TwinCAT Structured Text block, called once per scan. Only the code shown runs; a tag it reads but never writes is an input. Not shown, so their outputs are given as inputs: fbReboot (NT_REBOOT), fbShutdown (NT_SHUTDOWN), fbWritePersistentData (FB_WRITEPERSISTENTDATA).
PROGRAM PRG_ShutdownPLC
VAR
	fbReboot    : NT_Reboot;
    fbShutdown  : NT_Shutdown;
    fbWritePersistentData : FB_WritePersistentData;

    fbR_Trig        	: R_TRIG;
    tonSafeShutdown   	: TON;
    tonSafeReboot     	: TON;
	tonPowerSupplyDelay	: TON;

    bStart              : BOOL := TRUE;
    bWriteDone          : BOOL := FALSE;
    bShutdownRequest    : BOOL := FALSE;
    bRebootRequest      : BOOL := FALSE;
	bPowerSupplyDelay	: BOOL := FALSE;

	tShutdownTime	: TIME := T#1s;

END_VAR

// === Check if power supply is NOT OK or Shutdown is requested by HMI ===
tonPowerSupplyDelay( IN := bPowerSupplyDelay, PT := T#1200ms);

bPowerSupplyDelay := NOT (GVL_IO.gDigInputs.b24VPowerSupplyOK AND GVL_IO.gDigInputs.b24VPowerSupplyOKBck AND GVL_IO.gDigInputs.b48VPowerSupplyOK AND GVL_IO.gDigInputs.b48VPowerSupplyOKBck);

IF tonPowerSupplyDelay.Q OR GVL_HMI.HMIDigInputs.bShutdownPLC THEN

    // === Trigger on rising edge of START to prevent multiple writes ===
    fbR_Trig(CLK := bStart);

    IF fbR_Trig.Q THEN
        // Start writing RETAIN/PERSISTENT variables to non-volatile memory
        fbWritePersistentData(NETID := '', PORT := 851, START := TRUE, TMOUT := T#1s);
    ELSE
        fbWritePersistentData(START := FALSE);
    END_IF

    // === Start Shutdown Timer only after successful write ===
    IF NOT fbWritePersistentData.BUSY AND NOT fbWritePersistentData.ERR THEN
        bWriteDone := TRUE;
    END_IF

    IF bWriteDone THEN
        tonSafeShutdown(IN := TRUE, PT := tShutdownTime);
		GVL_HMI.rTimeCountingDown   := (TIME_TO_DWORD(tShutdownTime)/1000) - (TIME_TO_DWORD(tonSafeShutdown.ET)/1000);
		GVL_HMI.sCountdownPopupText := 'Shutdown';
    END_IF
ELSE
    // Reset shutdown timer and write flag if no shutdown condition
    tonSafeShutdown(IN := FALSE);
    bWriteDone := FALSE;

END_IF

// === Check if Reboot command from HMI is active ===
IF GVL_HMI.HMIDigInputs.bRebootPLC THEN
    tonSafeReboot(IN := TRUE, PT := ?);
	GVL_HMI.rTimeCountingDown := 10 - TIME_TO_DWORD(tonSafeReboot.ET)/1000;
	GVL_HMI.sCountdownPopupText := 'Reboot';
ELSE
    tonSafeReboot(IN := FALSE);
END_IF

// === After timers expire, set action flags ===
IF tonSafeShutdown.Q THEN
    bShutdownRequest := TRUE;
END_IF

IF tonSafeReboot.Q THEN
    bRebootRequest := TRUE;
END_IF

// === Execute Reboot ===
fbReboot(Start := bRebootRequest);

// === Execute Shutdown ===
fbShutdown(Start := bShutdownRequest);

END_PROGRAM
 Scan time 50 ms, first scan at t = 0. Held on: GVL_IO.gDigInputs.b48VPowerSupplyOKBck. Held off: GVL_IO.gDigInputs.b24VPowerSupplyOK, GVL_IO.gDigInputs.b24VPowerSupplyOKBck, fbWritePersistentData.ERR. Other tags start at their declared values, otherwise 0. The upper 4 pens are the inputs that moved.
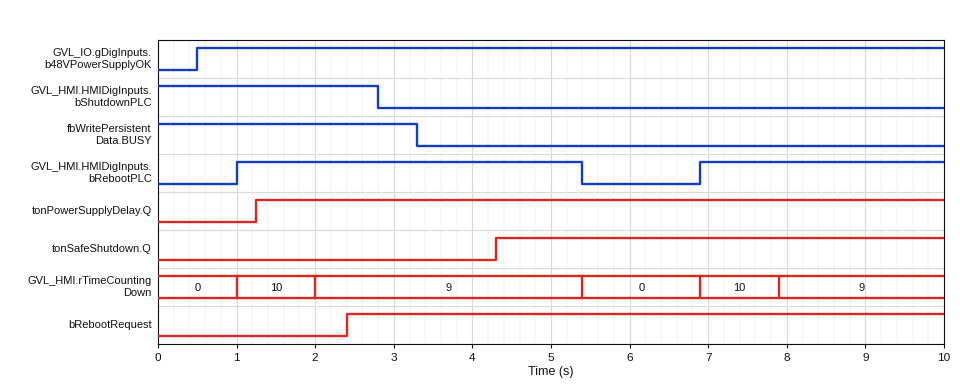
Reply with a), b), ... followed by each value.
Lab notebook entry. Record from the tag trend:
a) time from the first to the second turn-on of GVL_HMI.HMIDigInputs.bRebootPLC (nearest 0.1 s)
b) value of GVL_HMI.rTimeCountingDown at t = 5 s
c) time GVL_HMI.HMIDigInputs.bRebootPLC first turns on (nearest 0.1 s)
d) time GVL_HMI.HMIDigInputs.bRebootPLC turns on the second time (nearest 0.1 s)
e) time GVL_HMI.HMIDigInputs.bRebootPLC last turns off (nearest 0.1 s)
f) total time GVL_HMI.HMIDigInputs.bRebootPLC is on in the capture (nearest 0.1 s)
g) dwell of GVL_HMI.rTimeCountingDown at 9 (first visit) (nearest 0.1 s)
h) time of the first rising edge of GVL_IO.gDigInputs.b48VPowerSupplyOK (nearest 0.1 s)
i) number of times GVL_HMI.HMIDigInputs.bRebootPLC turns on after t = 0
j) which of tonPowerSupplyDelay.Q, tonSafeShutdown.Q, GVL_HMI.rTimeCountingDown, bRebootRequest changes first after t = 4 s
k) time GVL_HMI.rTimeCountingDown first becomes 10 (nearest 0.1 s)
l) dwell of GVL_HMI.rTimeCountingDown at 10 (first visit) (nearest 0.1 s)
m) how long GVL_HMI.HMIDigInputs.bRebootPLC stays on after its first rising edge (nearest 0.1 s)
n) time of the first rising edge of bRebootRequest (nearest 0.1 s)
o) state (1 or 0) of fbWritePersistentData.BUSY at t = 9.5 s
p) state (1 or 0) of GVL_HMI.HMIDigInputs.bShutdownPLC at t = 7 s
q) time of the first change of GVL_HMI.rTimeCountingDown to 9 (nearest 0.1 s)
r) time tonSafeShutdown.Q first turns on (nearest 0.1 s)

a) 5.9 s
b) 9
c) 1.0 s
d) 6.9 s
e) 5.4 s
f) 7.5 s
g) 3.4 s
h) 0.5 s
i) 2
j) tonSafeShutdown.Q
k) 1.0 s
l) 1.0 s
m) 4.4 s
n) 2.4 s
o) 0
p) 0
q) 2.0 s
r) 4.3 s
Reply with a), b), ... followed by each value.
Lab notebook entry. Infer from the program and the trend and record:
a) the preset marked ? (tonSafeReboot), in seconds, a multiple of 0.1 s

a) 1.4 s
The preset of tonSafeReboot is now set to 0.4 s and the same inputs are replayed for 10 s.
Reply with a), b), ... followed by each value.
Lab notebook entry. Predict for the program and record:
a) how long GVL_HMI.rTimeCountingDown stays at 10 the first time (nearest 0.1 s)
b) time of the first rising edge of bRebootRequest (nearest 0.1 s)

a) 4.4 s
b) 1.4 s
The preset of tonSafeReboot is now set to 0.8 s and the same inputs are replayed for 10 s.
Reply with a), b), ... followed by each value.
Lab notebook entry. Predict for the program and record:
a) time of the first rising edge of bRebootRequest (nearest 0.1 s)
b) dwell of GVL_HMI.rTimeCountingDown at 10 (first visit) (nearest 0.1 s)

a) 1.8 s
b) 4.4 s
